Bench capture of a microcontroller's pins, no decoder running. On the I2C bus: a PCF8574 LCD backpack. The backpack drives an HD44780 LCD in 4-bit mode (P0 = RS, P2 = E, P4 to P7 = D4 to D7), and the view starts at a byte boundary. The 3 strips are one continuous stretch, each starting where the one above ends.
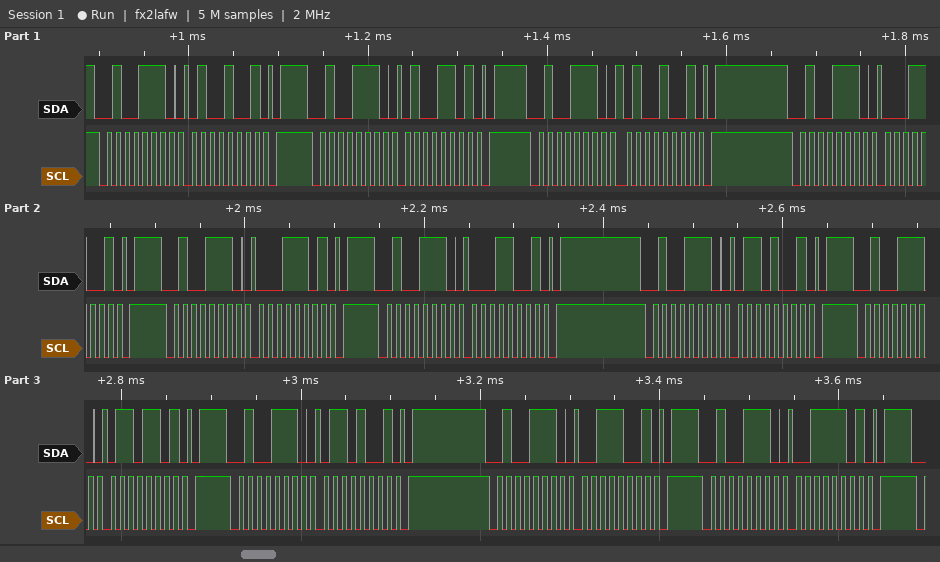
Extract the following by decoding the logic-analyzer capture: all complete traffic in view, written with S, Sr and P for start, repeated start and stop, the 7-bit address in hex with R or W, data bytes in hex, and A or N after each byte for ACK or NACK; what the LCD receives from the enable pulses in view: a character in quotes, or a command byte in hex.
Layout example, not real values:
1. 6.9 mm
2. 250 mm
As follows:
1. S 27W A 49 A P S 27W A 4D A P S 27W A 49 A P S 27W A 19 A P S 27W A 1D A P S 27W A 19 A P S 27W A 69 A P S 27W A 6D A P S 27W A 69 A P S 27W A 39 A P S 27W A 3D A P
2. 'A'
